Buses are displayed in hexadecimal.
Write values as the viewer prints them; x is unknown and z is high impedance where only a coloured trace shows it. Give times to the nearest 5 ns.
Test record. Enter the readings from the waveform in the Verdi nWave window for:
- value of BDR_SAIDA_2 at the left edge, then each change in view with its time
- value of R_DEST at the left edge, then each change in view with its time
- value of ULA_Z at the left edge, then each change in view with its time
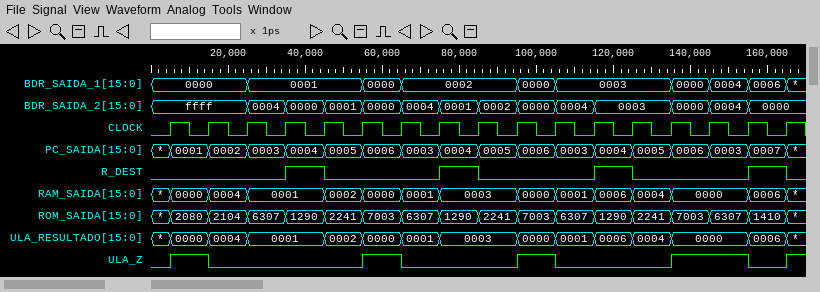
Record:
ffff, 0004 at 25 ns, 0000 at 35 ns, 0001 at 45 ns, 0000 at 55 ns, 0004 at 65 ns, 0001 at 75 ns, 0002 at 85 ns, 0000 at 95 ns, 0004 at 105 ns, 0003 at 115 ns, 0000 at 135 ns, 0004 at 145 ns, 0000 at 155 ns
0, 1 at 35 ns, 0 at 45 ns, 1 at 75 ns, 0 at 85 ns, 1 at 115 ns, 0 at 125 ns, 1 at 155 ns, 0 at 165 ns
0, 1 at 5 ns, 0 at 15 ns, 1 at 55 ns, 0 at 65 ns, 1 at 95 ns, 0 at 105 ns, 1 at 135 ns, 0 at 155 ns, 1 at 165 ns
